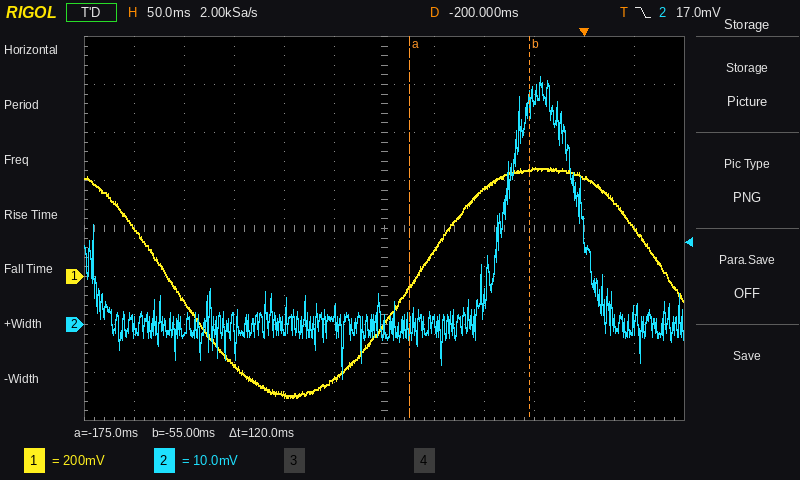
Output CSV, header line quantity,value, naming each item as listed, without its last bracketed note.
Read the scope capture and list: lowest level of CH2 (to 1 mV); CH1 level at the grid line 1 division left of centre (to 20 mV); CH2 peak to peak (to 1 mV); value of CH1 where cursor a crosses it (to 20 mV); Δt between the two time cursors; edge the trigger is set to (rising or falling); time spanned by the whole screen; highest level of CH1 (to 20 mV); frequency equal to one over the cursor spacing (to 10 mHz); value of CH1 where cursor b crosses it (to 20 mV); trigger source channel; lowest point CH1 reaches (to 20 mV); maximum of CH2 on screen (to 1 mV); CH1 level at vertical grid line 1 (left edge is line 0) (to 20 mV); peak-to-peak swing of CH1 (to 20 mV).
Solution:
quantity,value
lowest level of CH2,-11 mV
CH1 level at the grid line 1 division left of centre,-420 mV
CH2 peak to peak,63 mV
value of CH1 where cursor a crosses it,-40 mV
Δt between the two time cursors,120 ms
edge the trigger is set to,falling
time spanned by the whole screen,600 ms
highest level of CH1,460 mV
frequency equal to one over the cursor spacing,8.33 Hz
value of CH1 where cursor b crosses it,440 mV
trigger source channel,CH2
lowest point CH1 reaches,-500 mV
maximum of CH2 on screen,52 mV
CH1 level at vertical grid line 1 (left edge is line 0),200 mV
peak-to-peak swing of CH1,960 mV
